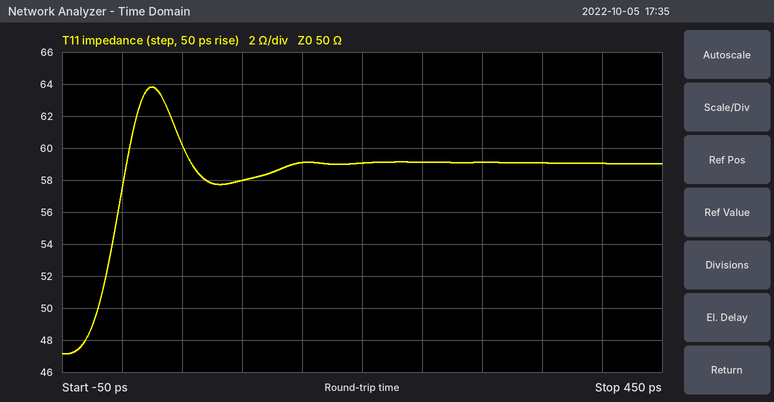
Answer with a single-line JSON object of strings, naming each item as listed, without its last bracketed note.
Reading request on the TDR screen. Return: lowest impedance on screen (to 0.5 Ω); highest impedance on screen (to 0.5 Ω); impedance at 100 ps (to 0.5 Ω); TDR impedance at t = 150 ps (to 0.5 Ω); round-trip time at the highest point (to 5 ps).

{"lowest impedance on screen": "47.0 Ω", "highest impedance on screen": "64.0 Ω", "impedance at 100 ps": "58.0 Ω", "TDR impedance at t = 150 ps": "59.0 Ω", "round-trip time at the highest point": "25 ps"}
